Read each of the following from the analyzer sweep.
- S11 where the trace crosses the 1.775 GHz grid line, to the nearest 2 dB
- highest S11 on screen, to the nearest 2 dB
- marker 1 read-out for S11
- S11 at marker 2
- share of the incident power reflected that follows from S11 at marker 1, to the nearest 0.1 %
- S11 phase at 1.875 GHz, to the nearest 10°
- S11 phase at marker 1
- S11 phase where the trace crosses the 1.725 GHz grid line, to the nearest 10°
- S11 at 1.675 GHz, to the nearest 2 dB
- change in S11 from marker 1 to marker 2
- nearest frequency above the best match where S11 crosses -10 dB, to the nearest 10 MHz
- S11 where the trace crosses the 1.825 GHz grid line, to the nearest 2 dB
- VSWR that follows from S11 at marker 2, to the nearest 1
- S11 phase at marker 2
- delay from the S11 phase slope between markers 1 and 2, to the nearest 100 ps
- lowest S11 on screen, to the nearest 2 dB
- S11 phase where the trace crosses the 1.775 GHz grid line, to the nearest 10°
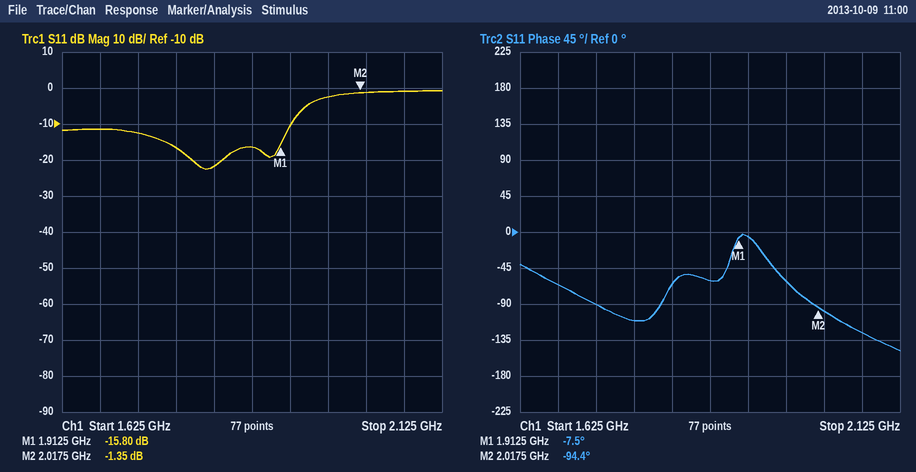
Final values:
-16 dB
0 dB
-15.80 dB
-1.35 dB
2.6 %
-60°
-7.5°
-90°
-12 dB
14.45 dB
1.93 GHz
-22 dB
13
-94.4°
2.3 ns
-22 dB
-110°
